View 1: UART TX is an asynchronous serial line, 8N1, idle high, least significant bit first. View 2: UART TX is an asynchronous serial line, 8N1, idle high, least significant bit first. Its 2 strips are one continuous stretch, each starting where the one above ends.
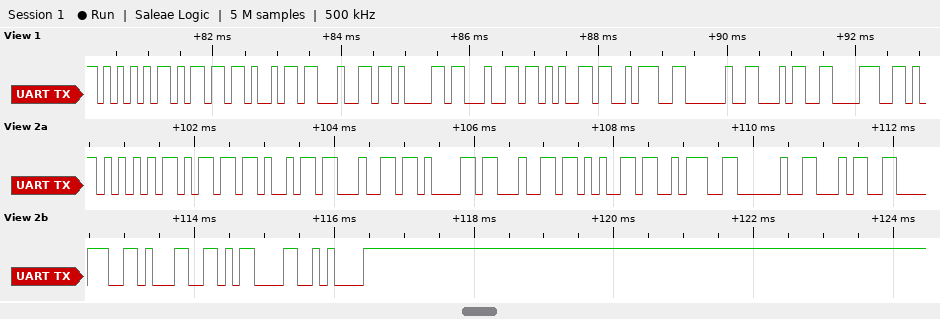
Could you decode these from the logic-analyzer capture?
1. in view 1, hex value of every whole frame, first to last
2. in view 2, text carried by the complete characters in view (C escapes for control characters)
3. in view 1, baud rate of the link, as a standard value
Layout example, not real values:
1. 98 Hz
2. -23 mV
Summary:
1. 0x55 0x6D 0x69 0x64 0x61 0x64 0x65 0x3A 0x20 0x34 0x38
2. "Umidade: 481\r\n"
3. 9600 baud
